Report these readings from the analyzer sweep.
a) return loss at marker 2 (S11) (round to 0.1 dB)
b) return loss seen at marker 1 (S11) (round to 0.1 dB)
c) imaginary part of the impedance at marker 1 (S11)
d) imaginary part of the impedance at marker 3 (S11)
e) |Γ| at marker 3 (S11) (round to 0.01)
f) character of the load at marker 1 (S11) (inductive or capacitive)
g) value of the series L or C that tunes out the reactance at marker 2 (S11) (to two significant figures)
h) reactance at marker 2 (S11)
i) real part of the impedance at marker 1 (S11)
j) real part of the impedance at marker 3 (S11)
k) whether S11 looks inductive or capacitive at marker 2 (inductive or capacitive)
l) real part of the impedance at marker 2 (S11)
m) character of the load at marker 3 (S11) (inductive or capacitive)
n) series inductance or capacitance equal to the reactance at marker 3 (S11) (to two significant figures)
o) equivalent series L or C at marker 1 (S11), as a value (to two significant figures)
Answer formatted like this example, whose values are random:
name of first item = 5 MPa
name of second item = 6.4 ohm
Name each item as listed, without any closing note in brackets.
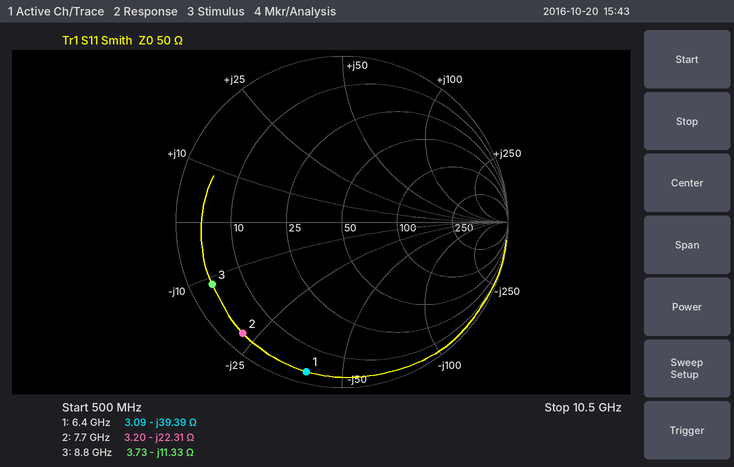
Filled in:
return loss at marker 2 (S11) = 0.9 dB
return loss seen at marker 1 (S11) = 0.7 dB
imaginary part of the impedance at marker 1 = -39.39 Ω
imaginary part of the impedance at marker 3 = -11.33 Ω
|Γ| at marker 3 (S11) = 0.87
character of the load at marker 1 (S11) = capacitive
value of the series L or C that tunes out the reactance at marker 2 (S11) = 460 pH
reactance at marker 2 = -22.31 Ω
real part of the impedance at marker 1 = 3.09 Ω
real part of the impedance at marker 3 = 3.73 Ω
whether S11 looks inductive or capacitive at marker 2 = capacitive
real part of the impedance at marker 2 = 3.20 Ω
character of the load at marker 3 (S11) = capacitive
series inductance or capacitance equal to the reactance at marker 3 (S11) = 1.6 pF
equivalent series L or C at marker 1 (S11), as a value = 630 fF
